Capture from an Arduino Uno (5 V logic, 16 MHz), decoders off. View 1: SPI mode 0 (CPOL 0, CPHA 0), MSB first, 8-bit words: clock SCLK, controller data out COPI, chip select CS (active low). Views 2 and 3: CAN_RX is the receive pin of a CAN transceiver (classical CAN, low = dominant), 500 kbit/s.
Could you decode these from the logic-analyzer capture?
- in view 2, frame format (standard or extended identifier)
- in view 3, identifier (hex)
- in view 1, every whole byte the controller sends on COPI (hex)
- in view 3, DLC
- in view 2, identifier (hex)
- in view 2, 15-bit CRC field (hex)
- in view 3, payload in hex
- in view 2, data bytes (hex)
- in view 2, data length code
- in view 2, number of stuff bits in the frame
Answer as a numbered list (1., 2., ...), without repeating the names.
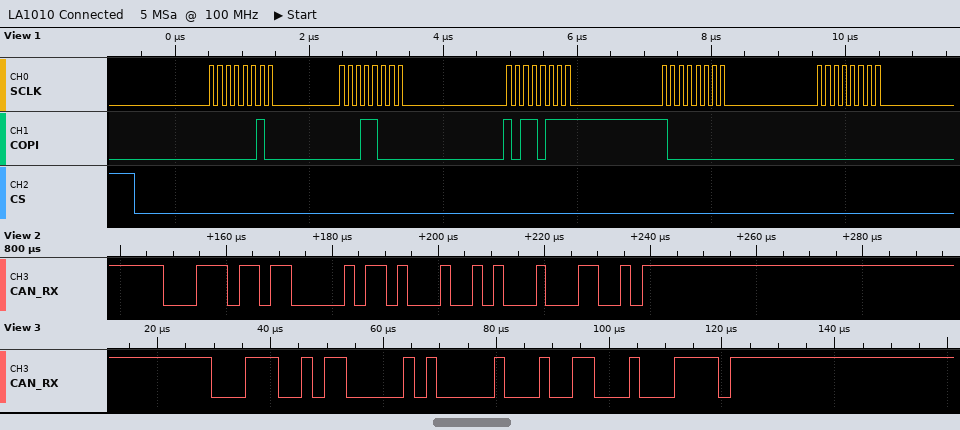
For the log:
1. standard
2. 0x1CB
3. 02 18 B7 80 00
4. 1
5. 0x1DB
6. 0x288C
7. 00
8. A2
9. 1
10. 1
